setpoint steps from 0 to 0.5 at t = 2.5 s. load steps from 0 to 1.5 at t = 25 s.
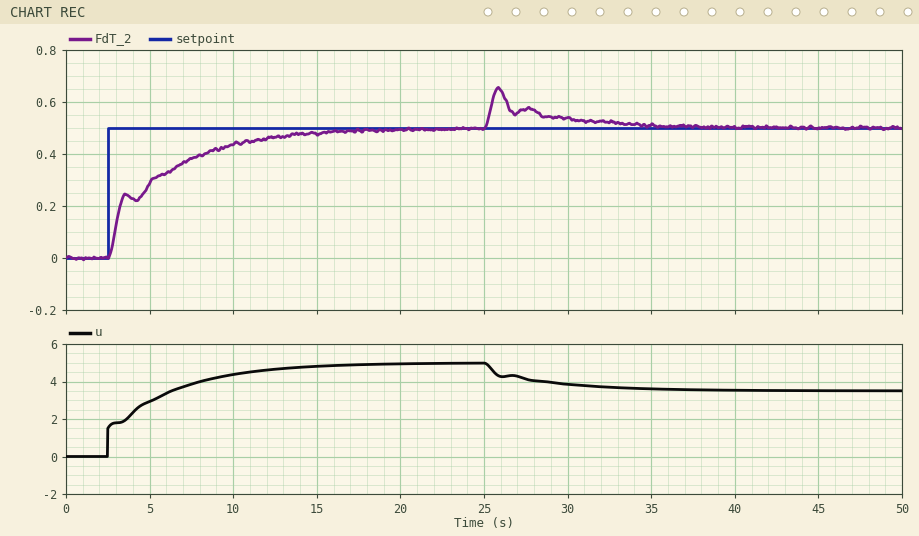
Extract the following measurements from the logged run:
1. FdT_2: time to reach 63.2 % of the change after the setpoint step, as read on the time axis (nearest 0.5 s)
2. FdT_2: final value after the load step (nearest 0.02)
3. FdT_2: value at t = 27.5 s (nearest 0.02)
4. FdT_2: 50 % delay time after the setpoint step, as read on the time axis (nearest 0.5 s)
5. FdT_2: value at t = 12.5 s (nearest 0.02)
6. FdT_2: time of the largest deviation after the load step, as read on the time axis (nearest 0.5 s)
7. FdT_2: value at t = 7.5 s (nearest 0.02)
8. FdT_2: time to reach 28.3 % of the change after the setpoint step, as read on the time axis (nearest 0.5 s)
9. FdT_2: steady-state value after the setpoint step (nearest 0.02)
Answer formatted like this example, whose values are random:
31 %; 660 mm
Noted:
5.5 s; 0.50; 0.58; 4.5 s; 0.46; 26.0 s; 0.38; 3.0 s; 0.50
